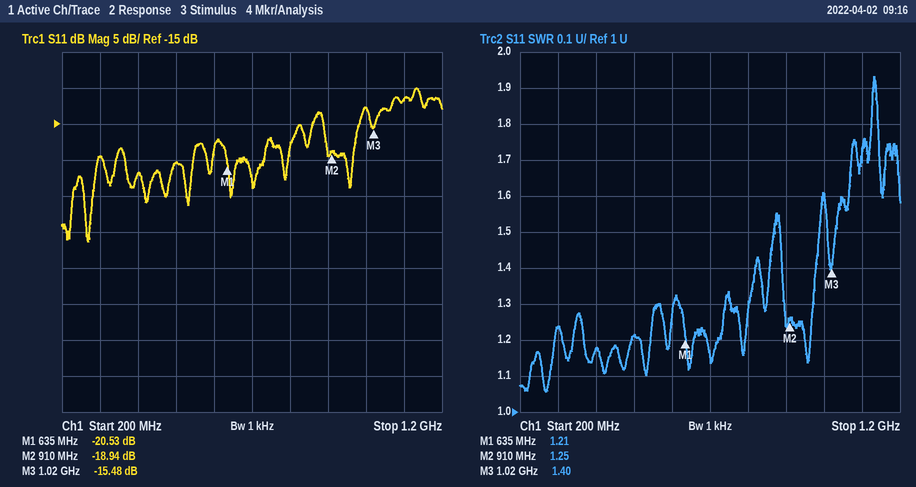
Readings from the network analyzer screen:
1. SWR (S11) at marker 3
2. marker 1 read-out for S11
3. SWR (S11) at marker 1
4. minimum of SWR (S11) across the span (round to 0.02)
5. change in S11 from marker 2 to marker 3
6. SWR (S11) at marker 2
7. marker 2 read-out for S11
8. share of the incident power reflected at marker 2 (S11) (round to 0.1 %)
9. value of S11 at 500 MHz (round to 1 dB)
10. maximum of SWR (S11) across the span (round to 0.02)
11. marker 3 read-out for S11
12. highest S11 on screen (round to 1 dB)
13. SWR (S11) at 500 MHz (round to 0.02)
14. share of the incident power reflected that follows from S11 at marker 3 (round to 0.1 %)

1.40
-20.53 dB
1.21
1.06
3.46 dB
1.25
-18.94 dB
1.3 %
-20 dB
1.94
-15.48 dB
-10 dB
1.22
2.8 %
